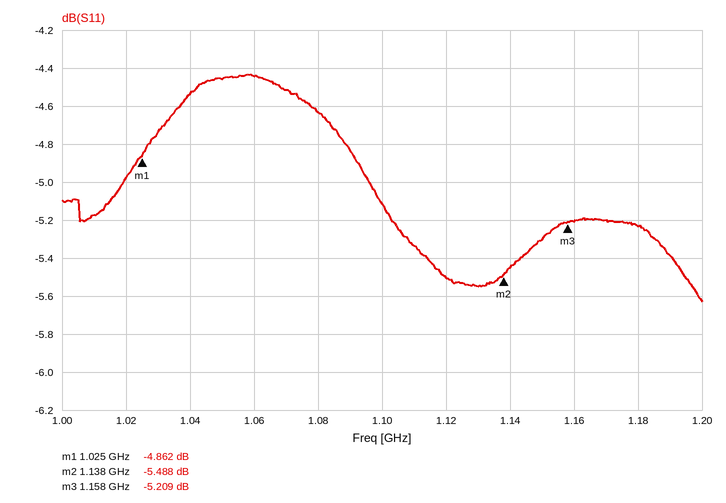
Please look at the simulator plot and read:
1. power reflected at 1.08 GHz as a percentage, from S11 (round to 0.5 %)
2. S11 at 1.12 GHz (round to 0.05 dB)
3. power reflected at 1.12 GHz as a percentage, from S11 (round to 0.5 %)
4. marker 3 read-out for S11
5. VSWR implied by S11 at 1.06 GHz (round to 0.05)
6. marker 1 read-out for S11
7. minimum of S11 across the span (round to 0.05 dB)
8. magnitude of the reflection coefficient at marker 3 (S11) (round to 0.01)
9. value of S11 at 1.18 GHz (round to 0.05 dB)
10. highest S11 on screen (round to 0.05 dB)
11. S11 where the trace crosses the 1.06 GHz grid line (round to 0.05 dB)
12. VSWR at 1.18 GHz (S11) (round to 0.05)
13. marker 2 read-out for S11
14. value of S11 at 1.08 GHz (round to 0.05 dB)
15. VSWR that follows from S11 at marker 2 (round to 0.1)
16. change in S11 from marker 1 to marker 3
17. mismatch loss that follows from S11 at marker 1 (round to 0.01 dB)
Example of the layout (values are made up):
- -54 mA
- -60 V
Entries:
- 34.5 %
- -5.50 dB
- 28.0 %
- -5.209 dB
- 4.00
- -4.862 dB
- -5.65 dB
- 0.55
- -5.25 dB
- -4.45 dB
- -4.45 dB
- 3.40
- -5.488 dB
- -4.65 dB
- 3.3
- -0.347 dB
- 1.72 dB
